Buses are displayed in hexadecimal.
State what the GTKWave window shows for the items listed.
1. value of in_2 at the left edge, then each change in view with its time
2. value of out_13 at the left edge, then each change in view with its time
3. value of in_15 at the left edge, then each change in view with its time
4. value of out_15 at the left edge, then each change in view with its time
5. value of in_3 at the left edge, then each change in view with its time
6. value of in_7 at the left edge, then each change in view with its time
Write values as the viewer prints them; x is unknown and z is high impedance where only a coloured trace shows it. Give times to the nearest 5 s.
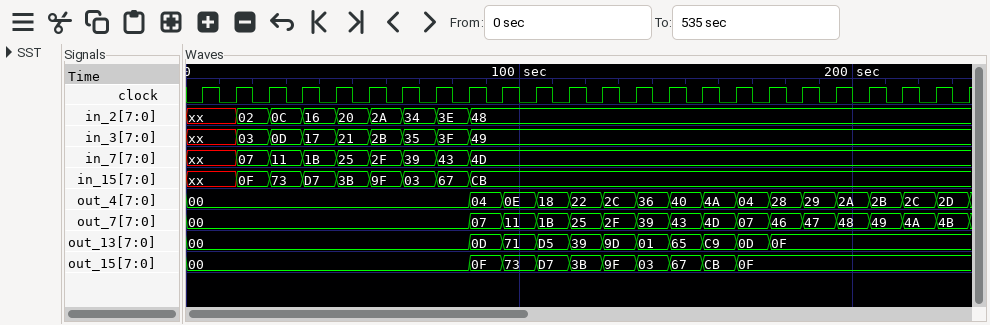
xx, 02 at 15 s, 0C at 25 s, 16 at 35 s, 20 at 45 s, 2A at 55 s, 34 at 65 s, 3E at 75 s, 48 at 85 s
00, 0D at 85 s, 71 at 95 s, D5 at 105 s, 39 at 115 s, 9D at 125 s, 01 at 135 s, 65 at 145 s, C9 at 155 s, 0D at 165 s, 0F at 175 s
xx, 0F at 15 s, 73 at 25 s, D7 at 35 s, 3B at 45 s, 9F at 55 s, 03 at 65 s, 67 at 75 s, CB at 85 s
00, 0F at 85 s, 73 at 95 s, D7 at 105 s, 3B at 115 s, 9F at 125 s, 03 at 135 s, 67 at 145 s, CB at 155 s, 0F at 165 s
xx, 03 at 15 s, 0D at 25 s, 17 at 35 s, 21 at 45 s, 2B at 55 s, 35 at 65 s, 3F at 75 s, 49 at 85 s
xx, 07 at 15 s, 11 at 25 s, 1B at 35 s, 25 at 45 s, 2F at 55 s, 39 at 65 s, 43 at 75 s, 4D at 85 s
